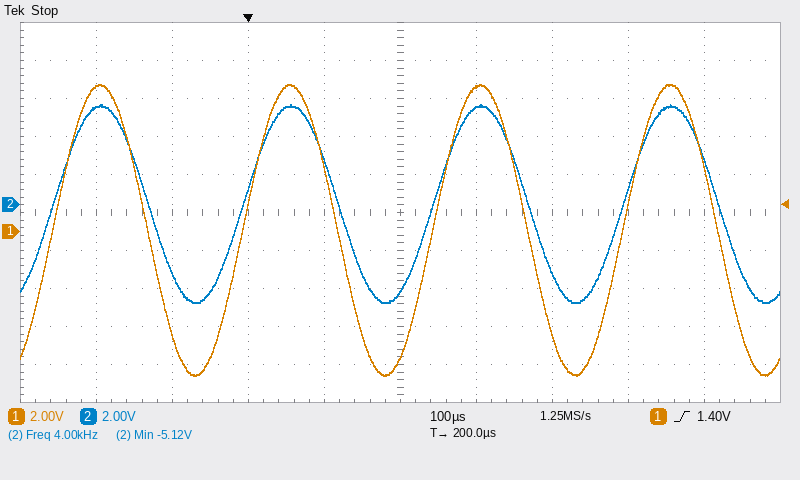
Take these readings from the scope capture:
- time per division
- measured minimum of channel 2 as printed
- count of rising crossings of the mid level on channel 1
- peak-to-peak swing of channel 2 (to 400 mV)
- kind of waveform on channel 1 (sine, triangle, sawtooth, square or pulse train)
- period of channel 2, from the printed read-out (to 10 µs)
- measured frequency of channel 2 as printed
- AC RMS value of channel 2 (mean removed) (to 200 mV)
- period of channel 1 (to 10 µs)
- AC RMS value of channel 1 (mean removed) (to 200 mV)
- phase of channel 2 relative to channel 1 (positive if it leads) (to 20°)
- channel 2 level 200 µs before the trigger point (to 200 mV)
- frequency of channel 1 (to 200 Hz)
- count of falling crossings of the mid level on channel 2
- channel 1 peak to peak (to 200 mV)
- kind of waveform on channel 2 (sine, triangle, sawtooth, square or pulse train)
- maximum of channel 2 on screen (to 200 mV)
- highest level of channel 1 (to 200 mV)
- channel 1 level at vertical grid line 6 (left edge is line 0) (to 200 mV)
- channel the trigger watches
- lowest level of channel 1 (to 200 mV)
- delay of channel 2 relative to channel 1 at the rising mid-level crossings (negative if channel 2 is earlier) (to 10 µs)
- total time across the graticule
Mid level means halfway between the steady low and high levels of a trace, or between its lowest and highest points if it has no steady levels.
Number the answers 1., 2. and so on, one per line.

1. 100 µs
2. -5.12 V
3. 4
4. 10.4 V
5. sine
6. 250 µs
7. 4.00 kHz
8. 3.6 V
9. 250 µs
10. 5.4 V
11. 0°
12. 5.2 V
13. 4.0 kHz
14. 4
15. 15.4 V
16. sine
17. 5.2 V
18. 7.8 V
19. 7.6 V
20. channel 1
21. -7.6 V
22. 0 µs
23. 1 ms
